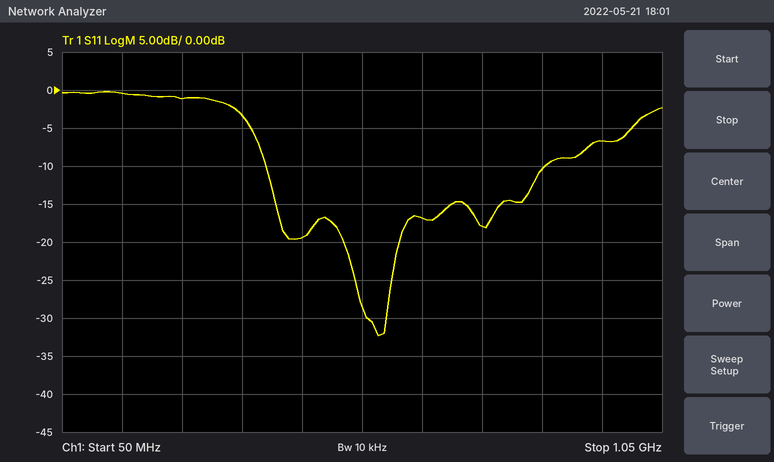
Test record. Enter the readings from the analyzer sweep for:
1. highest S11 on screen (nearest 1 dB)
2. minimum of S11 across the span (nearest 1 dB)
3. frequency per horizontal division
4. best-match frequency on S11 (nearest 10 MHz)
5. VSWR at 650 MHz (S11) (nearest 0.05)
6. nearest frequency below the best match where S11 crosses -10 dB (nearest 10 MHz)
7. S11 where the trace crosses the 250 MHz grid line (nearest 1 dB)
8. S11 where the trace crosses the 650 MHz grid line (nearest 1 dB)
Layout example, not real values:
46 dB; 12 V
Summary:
0 dB; -32 dB; 100 MHz; 580 MHz; 1.35; 390 MHz; -1 dB; -17 dB
